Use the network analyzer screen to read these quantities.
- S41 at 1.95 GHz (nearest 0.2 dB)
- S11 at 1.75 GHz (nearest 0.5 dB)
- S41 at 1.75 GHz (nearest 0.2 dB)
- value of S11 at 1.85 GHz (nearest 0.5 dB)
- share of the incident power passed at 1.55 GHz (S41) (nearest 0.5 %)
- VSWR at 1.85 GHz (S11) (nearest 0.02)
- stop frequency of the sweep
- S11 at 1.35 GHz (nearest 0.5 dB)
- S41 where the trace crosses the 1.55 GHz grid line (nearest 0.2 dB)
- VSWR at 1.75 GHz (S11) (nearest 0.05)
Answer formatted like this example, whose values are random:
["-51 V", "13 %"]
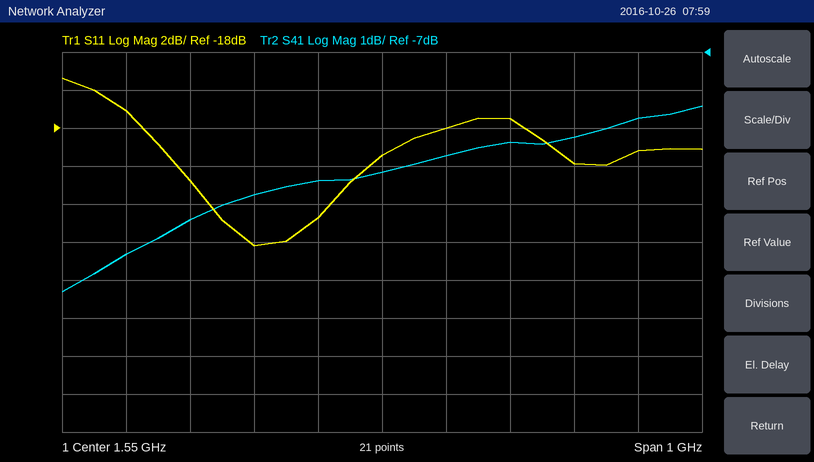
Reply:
["-8.8 dB", "-17.5 dB", "-9.4 dB", "-20.0 dB", "9.5 %", "1.22", "2.05 GHz", "-24.0 dB", "-10.2 dB", "1.30"]
